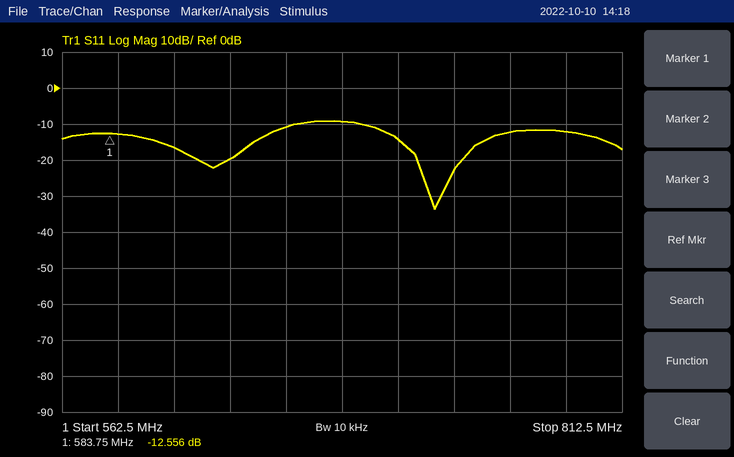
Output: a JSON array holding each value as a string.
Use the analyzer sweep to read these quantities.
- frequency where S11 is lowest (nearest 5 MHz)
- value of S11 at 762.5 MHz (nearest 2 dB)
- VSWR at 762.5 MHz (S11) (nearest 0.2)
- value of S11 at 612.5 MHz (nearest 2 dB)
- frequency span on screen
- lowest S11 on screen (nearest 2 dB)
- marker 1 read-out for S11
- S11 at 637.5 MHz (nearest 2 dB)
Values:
["730 MHz", "-12 dB", "1.6", "-16 dB", "250 MHz", "-34 dB", "-12.556 dB", "-20 dB"]
